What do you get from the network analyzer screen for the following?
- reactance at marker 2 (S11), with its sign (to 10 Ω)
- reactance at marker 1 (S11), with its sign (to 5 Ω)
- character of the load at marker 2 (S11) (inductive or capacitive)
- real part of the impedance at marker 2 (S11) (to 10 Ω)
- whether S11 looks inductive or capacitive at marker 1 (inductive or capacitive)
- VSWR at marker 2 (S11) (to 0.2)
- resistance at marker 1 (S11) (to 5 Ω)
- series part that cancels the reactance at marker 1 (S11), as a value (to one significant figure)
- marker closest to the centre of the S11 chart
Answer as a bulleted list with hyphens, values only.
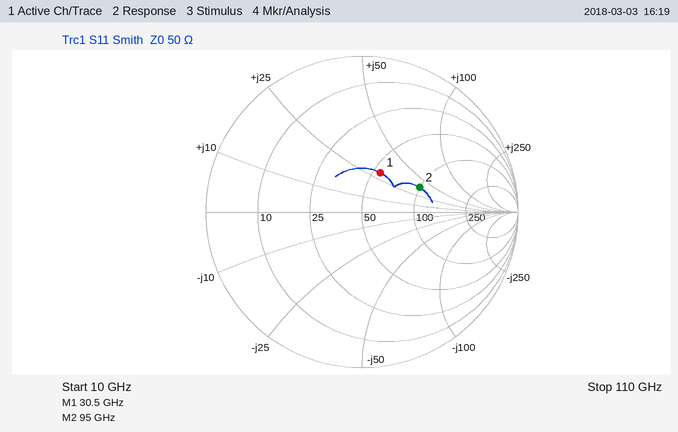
- +40 Ω
- +30 Ω
- inductive
- 100 Ω
- inductive
- 2.4
- 55 Ω
- 200 fF
- marker 1
